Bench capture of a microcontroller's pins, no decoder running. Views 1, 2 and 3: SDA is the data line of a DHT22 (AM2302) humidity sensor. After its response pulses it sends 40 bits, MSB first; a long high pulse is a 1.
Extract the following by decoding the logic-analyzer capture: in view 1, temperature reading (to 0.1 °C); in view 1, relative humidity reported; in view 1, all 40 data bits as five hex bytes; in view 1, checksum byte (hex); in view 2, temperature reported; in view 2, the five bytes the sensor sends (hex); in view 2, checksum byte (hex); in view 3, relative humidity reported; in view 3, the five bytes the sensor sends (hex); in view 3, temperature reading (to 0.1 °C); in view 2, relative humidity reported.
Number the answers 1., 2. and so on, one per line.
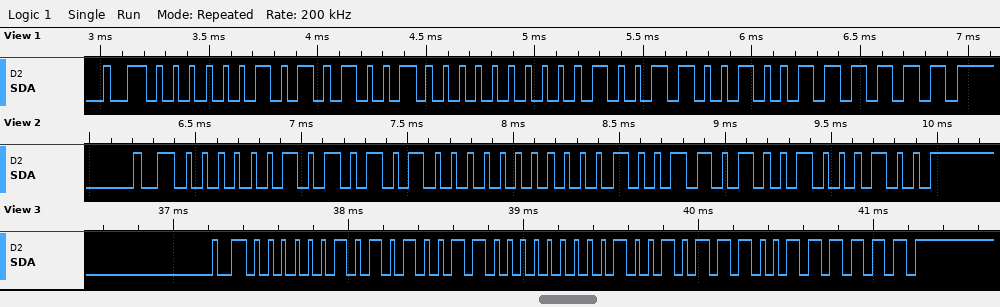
1. 15.3 °C
2. 67.6 %
3. 02 A4 00 99 3F
4. 0x3F
5. 15.4 °C
6. 02 A8 00 9A 44
7. 0x44
8. 67.8 %
9. 02 A6 00 97 3F
10. 15.1 °C
11. 68.0 %
